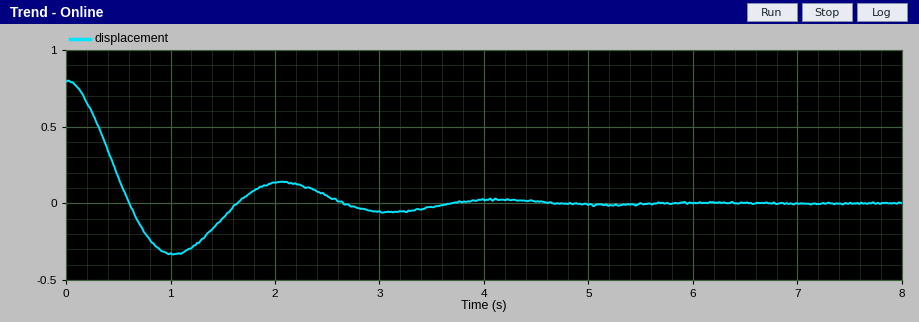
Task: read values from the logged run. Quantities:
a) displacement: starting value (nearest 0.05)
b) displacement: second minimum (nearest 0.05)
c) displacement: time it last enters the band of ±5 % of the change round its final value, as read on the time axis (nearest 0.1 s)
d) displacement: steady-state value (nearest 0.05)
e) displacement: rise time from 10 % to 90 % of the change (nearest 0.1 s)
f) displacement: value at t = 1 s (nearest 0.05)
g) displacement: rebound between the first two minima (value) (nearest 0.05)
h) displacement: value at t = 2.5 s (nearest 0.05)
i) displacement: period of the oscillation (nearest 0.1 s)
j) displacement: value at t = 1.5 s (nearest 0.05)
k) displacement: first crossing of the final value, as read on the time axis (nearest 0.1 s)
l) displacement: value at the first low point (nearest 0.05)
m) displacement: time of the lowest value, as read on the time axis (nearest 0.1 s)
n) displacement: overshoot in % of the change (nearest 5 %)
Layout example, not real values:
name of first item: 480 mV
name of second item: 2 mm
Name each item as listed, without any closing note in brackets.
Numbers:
displacement: starting value: 0.80
displacement: second minimum: -0.05
displacement: time it last enters the band of ±5 % of the change round its final value, as read on the time axis: 3.4 s
displacement: steady-state value: 0.00
displacement: rise time from 10 % to 90 % of the change: 0.4 s
displacement: value at t = 1 s: -0.35
displacement: rebound between the first two minima (value): 0.15
displacement: value at t = 2.5 s: 0.05
displacement: period of the oscillation: 2.1 s
displacement: value at t = 1.5 s: -0.10
displacement: first crossing of the final value, as read on the time axis: 0.6 s
displacement: value at the first low point: -0.35
displacement: time of the lowest value, as read on the time axis: 1.0 s
displacement: overshoot in % of the change: 40 %
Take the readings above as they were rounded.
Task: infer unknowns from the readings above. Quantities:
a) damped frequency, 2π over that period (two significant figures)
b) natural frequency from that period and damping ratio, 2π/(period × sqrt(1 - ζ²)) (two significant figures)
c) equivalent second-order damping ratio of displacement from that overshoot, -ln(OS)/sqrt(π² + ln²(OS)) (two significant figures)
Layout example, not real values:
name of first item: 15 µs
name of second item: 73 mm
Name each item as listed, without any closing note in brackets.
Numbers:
damped frequency, 2π over that period: 3.0 rad/s
natural frequency from that period and damping ratio, 2π/(period × sqrt(1 - ζ²)): 3.1 rad/s
equivalent second-order damping ratio of displacement from that overshoot, -ln(OS)/sqrt(π² + ln²(OS)): 0.28
